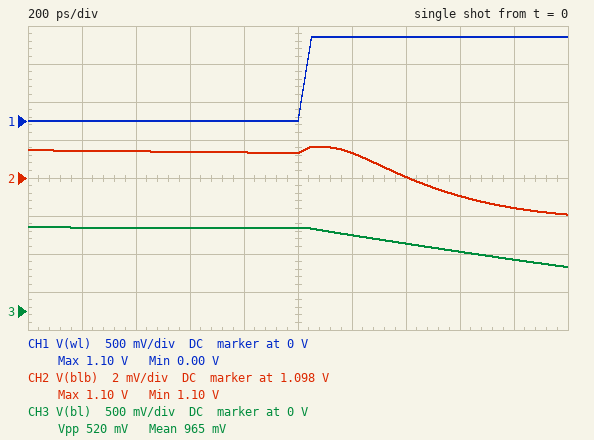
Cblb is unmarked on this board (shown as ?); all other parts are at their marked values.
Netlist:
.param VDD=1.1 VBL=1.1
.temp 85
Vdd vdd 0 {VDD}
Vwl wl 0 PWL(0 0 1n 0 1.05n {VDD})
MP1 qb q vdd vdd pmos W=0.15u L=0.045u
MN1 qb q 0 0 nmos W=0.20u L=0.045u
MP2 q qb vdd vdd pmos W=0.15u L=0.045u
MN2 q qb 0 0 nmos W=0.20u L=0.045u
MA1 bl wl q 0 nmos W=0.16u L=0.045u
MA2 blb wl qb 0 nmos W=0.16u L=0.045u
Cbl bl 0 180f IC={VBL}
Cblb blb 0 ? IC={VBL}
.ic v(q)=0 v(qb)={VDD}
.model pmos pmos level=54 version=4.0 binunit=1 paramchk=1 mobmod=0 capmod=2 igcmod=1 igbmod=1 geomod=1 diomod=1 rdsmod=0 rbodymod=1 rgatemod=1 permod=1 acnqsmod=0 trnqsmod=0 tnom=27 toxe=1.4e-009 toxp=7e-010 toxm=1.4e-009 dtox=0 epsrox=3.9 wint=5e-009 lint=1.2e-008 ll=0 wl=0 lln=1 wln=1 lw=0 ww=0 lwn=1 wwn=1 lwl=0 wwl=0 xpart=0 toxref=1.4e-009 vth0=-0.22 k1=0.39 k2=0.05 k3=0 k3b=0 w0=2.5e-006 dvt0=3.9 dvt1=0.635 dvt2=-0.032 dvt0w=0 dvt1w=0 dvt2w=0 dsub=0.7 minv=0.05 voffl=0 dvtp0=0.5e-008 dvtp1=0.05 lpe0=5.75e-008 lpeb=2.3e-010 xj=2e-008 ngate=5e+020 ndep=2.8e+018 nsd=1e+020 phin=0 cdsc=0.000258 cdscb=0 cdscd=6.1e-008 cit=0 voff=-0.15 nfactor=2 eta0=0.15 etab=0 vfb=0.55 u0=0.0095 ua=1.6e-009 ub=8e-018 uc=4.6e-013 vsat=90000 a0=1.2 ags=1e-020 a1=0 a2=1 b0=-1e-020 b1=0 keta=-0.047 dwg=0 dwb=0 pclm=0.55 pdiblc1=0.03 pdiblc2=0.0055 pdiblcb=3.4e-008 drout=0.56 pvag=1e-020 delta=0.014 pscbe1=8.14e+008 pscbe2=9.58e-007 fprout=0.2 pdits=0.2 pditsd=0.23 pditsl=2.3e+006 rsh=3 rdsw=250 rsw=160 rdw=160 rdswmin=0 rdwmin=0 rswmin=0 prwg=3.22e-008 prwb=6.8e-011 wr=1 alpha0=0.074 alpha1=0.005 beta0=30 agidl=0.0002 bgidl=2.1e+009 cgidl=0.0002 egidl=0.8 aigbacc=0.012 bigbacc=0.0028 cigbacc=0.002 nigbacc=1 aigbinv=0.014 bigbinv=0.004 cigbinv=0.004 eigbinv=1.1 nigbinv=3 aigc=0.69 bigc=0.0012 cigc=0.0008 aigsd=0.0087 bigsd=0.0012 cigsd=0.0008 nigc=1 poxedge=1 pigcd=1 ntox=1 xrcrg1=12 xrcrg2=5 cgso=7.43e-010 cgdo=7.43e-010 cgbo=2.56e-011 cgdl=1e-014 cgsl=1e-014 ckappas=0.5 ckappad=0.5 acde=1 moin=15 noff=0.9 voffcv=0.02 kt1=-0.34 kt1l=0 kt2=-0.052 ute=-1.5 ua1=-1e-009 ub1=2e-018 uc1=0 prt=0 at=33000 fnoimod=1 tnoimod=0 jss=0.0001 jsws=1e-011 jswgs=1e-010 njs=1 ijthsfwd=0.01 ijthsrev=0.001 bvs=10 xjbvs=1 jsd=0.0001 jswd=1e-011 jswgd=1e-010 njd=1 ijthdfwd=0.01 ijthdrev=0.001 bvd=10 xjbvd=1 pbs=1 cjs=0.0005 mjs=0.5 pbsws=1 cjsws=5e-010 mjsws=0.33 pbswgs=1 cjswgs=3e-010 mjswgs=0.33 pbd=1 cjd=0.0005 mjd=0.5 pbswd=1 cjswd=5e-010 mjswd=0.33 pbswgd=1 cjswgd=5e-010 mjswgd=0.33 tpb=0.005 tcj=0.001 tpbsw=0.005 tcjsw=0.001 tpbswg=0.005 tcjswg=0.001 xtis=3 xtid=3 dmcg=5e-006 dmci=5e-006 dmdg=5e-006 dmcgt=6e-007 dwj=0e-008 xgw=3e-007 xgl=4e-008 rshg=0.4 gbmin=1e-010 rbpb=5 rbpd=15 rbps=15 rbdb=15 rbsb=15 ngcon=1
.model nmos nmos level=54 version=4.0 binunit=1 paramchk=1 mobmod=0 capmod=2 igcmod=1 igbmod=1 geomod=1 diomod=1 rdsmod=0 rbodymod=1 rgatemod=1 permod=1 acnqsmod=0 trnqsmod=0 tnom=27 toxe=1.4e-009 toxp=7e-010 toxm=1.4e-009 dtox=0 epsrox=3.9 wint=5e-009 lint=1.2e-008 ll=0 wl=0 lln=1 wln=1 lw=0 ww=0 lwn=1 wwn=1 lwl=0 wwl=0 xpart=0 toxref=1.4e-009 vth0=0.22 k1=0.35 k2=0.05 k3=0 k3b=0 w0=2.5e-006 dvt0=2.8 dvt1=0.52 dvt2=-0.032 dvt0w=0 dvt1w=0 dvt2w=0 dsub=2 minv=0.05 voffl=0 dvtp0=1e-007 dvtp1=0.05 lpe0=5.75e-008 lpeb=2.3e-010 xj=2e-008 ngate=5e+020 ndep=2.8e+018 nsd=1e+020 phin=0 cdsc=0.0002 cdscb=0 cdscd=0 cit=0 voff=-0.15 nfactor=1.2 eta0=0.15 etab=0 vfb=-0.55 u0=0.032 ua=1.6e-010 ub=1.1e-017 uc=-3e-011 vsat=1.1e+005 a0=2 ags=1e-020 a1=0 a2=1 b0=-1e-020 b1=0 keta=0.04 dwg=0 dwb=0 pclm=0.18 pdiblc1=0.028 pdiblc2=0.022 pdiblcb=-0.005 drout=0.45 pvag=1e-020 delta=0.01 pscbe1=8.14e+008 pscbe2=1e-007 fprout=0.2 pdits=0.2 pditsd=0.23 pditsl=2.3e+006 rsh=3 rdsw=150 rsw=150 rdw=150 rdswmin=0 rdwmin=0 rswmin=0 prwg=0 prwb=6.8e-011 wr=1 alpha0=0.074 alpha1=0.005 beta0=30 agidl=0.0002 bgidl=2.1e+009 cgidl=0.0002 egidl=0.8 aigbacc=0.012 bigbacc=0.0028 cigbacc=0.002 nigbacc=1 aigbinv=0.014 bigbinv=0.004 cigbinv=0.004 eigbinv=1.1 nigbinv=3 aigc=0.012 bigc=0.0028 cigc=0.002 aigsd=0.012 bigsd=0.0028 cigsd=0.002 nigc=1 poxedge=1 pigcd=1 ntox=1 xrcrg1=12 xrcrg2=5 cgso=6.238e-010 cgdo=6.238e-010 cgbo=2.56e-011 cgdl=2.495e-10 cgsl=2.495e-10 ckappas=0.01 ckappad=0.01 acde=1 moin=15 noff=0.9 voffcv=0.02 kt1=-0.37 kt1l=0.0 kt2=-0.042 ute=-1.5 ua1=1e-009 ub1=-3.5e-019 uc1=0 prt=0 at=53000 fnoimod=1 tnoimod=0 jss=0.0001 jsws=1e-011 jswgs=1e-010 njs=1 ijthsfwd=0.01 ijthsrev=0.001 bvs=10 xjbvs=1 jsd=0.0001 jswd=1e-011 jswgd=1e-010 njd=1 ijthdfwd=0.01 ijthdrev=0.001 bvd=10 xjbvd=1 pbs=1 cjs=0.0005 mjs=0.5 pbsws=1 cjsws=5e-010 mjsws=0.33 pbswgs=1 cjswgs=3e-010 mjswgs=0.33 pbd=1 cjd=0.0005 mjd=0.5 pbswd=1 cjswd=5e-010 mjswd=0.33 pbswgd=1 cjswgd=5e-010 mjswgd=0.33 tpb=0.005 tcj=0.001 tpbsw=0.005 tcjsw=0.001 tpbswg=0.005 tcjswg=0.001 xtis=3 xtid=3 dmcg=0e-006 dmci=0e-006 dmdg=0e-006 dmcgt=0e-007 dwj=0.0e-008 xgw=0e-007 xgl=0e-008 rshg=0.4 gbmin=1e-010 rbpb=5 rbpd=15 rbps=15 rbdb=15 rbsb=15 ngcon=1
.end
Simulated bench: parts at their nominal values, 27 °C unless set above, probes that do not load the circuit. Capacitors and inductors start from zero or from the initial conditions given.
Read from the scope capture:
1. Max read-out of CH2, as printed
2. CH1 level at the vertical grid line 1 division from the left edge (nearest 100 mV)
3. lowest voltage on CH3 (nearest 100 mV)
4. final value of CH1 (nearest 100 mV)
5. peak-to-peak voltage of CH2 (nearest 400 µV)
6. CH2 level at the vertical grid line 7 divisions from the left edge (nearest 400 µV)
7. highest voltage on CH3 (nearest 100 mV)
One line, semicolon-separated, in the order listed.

1.10 V; 0 V; 600 mV; 1.1 V; 3.6 mV; 1.0980 V; 1.1 V
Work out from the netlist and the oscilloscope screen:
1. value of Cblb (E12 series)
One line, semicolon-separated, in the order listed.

390 fF
